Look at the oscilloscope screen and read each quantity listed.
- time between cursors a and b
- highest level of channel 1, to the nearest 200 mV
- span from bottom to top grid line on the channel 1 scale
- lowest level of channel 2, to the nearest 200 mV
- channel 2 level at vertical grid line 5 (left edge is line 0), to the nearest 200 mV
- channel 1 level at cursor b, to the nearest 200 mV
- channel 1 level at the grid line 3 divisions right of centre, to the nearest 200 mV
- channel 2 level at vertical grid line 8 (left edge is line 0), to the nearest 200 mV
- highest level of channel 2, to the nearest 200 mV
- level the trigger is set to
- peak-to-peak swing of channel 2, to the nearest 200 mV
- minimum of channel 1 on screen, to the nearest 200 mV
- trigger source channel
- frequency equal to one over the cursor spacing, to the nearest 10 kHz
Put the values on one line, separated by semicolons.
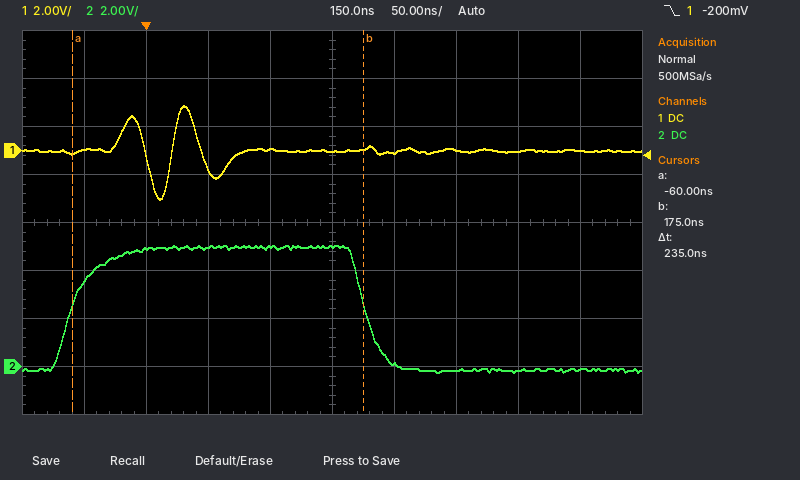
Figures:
235 ns; 1.8 V; 16 V; -200 mV; 5.0 V; 0.0 V; 0.0 V; -200 mV; 5.0 V; -200 mV; 5.2 V; -2.0 V; channel 1; 4.26 MHz
